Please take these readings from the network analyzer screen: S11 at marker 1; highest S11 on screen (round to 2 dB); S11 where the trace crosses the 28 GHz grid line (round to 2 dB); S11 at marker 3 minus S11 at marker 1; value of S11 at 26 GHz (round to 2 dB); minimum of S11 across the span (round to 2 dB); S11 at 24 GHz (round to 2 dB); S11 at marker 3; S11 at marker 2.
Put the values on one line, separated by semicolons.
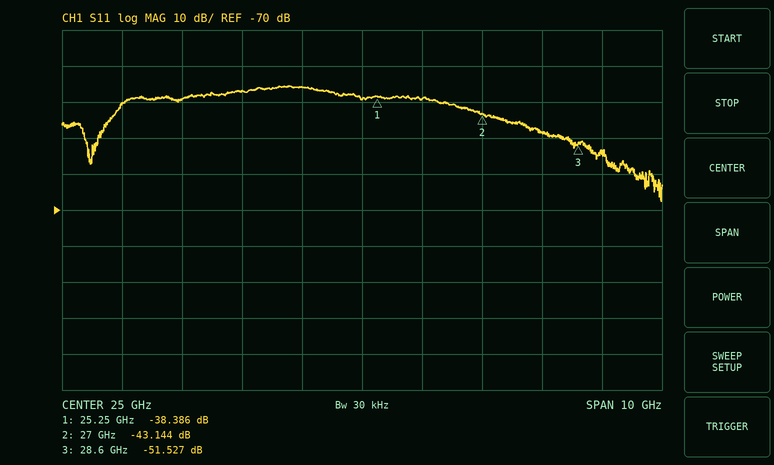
-38.386 dB; -36 dB; -48 dB; -13.141 dB; -40 dB; -68 dB; -36 dB; -51.527 dB; -43.144 dB
